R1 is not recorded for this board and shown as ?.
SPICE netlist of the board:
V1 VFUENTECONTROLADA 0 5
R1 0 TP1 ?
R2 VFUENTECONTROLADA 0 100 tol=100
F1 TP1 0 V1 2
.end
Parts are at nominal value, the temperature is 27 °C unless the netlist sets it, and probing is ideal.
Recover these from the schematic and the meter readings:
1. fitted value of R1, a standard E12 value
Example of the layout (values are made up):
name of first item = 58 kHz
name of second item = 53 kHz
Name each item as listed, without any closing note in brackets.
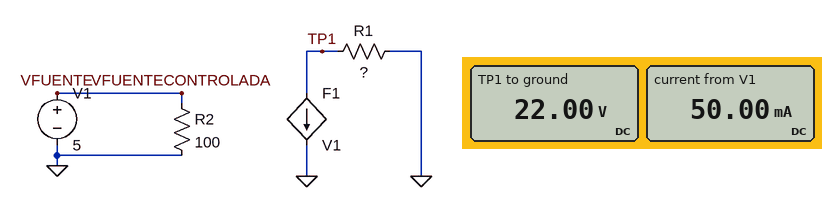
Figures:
fitted value of R1, a standard E12 value = 220 Ω
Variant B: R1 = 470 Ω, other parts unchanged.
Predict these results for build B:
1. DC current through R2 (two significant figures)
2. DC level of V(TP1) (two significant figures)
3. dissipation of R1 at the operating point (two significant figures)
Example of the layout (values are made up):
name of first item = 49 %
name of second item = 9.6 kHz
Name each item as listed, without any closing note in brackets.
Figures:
DC current through R2 = 50 mA
DC level of V(TP1) = 47 V
dissipation of R1 at the operating point = 4.7 W
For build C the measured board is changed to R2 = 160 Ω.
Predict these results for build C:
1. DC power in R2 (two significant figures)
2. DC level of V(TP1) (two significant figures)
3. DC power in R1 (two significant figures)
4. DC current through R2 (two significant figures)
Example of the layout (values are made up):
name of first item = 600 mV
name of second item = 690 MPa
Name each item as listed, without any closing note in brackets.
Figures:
DC power in R2 = 160 mW
DC level of V(TP1) = 14 V
DC power in R1 = 860 mW
DC current through R2 = 31 mA
